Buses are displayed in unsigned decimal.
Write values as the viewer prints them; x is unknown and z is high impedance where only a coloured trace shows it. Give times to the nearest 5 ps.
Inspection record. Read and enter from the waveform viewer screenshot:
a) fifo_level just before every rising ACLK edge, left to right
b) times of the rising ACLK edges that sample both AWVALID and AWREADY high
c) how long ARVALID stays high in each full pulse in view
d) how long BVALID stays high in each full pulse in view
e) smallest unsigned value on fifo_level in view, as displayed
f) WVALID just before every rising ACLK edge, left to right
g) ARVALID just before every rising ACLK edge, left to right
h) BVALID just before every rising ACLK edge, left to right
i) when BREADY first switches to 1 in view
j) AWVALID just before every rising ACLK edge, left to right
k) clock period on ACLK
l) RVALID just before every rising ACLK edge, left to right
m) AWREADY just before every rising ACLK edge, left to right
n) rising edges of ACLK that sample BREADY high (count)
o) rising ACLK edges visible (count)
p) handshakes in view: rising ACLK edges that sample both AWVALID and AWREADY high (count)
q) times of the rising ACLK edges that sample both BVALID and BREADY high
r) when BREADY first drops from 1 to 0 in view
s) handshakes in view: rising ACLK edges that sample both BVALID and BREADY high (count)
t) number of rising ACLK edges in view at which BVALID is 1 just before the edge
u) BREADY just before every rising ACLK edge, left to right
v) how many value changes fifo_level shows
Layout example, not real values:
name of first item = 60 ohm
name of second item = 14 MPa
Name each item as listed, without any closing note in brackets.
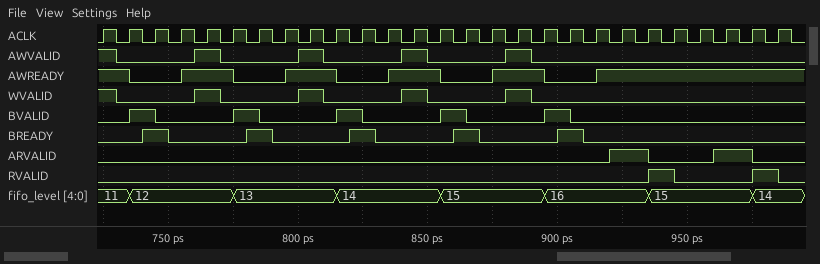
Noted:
fifo_level just before every rising ACLK edge, left to right = 11, 11, 12, 12, 12, 12, 13, 13, 13, 13, 14, 14, 14, 14, 15, 15, 15, 15, 16, 16, 16, 16, 15, 15, 15, 15, 14
times of the rising ACLK edges that sample both AWVALID and AWREADY high = 725 ps, 765 ps, 805 ps, 845 ps, 885 ps
how long ARVALID stays high in each full pulse in view = 15 ps, 15 ps
how long BVALID stays high in each full pulse in view = 10 ps, 10 ps, 10 ps, 10 ps, 10 ps
smallest unsigned value on fifo_level in view, as displayed = 11
WVALID just before every rising ACLK edge, left to right = 1 0 0 0 1 0 0 0 1 0 0 0 1 0 0 0 1 0 0 0 0 0 0 0 0 0 0
ARVALID just before every rising ACLK edge, left to right = 0 0 0 0 0 0 0 0 0 0 0 0 0 0 0 0 0 0 0 0 1 1 0 0 1 1 0
BVALID just before every rising ACLK edge, left to right = 0 0 1 0 0 0 1 0 0 0 1 0 0 0 1 0 0 0 1 0 0 0 0 0 0 0 0
when BREADY first switches to 1 in view = 740 ps
AWVALID just before every rising ACLK edge, left to right = 1 0 0 0 1 0 0 0 1 0 0 0 1 0 0 0 1 0 0 0 0 0 0 0 0 0 0
clock period on ACLK = 10 ps
RVALID just before every rising ACLK edge, left to right = 0 0 0 0 0 0 0 0 0 0 0 0 0 0 0 0 0 0 0 0 0 0 1 0 0 0 1
AWREADY just before every rising ACLK edge, left to right = 1 1 0 0 1 1 0 0 1 1 0 0 1 1 0 0 1 1 0 0 1 1 1 1 1 1 1
rising edges of ACLK that sample BREADY high = 5
rising ACLK edges visible = 27
handshakes in view: rising ACLK edges that sample both AWVALID and AWREADY high = 5
times of the rising ACLK edges that sample both BVALID and BREADY high = 745 ps, 785 ps, 825 ps, 865 ps, 905 ps
when BREADY first drops from 1 to 0 in view = 750 ps
handshakes in view: rising ACLK edges that sample both BVALID and BREADY high = 5
number of rising ACLK edges in view at which BVALID is 1 just before the edge = 5
BREADY just before every rising ACLK edge, left to right = 0 0 1 0 0 0 1 0 0 0 1 0 0 0 1 0 0 0 1 0 0 0 0 0 0 0 0
how many value changes fifo_level shows = 7
